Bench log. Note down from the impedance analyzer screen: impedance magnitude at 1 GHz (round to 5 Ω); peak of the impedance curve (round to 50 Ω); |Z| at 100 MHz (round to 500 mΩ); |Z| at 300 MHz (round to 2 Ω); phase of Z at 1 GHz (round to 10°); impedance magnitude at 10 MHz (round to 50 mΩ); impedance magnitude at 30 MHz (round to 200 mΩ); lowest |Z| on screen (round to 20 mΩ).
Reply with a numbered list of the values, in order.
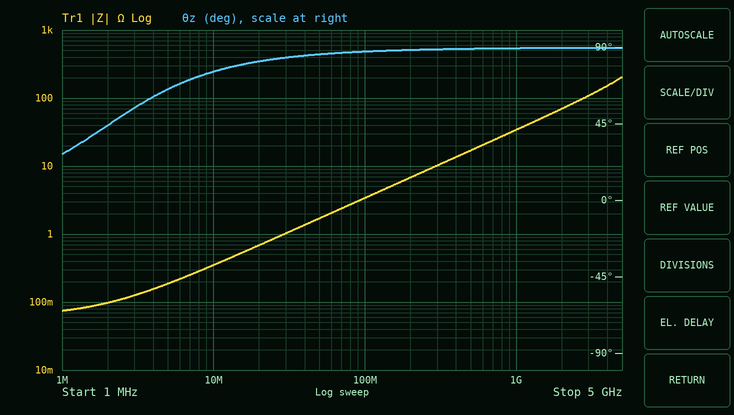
1. 35 Ω
2. 200 Ω
3. 3.5 Ω
4. 10 Ω
5. 90°
6. 350 mΩ
7. 1.0 Ω
8. 80 mΩ
